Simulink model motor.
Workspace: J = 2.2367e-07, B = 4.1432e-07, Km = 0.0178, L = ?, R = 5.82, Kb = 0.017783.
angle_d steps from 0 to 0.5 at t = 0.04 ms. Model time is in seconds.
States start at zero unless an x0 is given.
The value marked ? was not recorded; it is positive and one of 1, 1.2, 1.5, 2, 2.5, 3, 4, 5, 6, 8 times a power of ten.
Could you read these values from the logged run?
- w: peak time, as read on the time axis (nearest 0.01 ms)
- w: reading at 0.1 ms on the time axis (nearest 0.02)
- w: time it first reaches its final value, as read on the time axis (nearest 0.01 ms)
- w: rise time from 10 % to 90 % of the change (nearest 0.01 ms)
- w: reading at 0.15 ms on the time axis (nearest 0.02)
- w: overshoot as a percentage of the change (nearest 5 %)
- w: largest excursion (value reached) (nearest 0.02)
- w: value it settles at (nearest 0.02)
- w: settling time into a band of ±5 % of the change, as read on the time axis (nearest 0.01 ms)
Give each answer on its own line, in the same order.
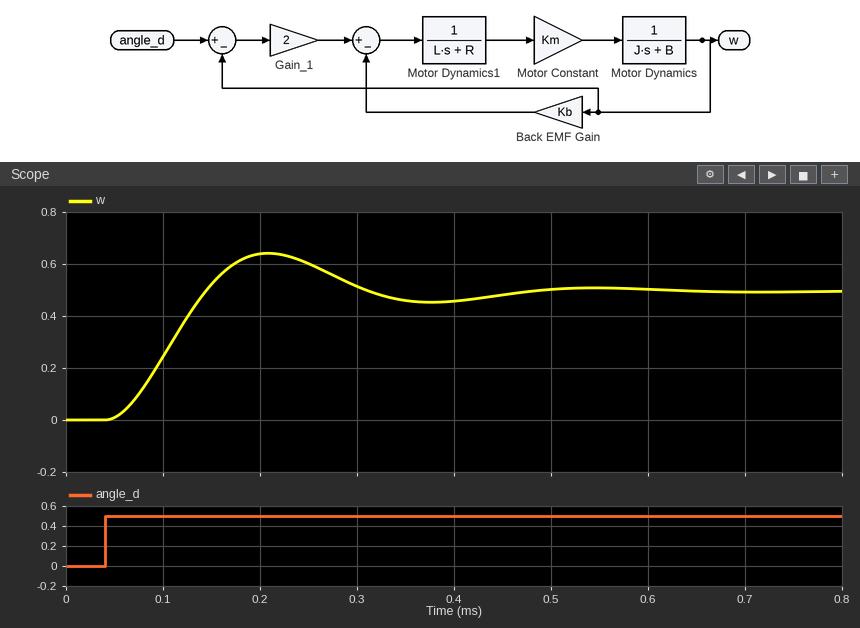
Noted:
0.21 ms
0.24
0.14 ms
0.07 ms
0.52
30 %
0.64
0.50
0.43 ms
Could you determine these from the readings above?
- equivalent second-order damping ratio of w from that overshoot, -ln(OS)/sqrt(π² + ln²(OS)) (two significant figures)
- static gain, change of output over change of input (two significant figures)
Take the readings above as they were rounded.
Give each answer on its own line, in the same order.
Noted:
0.36
1.0
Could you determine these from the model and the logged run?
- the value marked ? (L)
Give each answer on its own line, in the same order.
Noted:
0.0004
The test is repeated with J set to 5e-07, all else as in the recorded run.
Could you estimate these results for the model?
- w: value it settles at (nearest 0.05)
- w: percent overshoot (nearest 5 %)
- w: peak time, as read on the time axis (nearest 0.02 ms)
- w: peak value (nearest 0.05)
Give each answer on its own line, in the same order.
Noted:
0.50
15 %
0.32 ms
0.55
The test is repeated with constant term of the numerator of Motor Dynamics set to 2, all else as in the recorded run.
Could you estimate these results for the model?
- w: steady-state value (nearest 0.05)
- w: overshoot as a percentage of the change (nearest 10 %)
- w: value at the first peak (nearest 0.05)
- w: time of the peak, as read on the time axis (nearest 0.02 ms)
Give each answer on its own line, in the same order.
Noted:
0.50
40 %
0.70
0.16 ms
